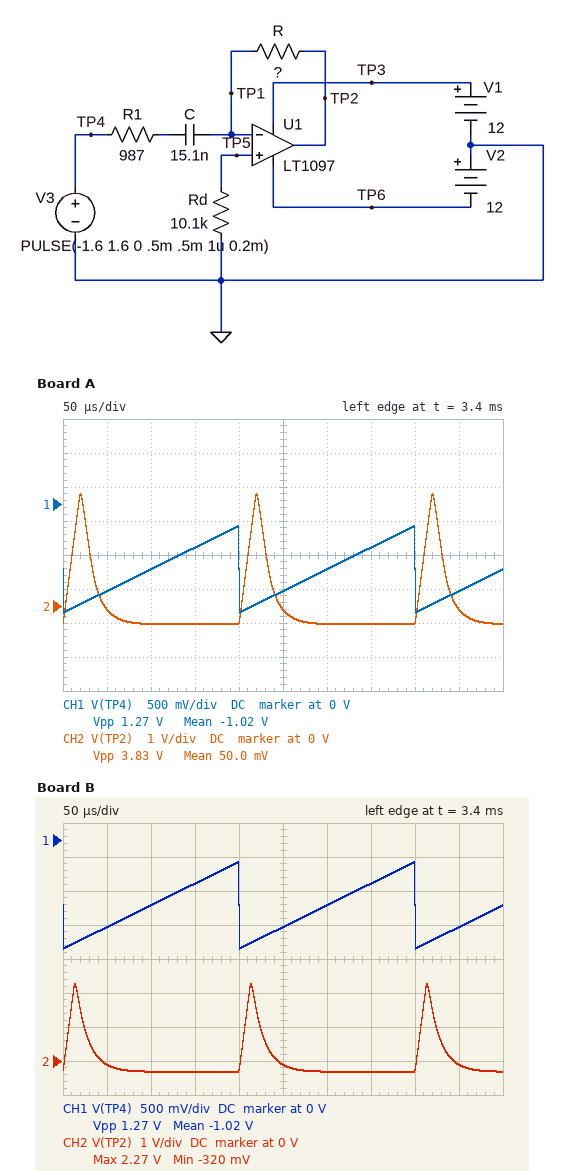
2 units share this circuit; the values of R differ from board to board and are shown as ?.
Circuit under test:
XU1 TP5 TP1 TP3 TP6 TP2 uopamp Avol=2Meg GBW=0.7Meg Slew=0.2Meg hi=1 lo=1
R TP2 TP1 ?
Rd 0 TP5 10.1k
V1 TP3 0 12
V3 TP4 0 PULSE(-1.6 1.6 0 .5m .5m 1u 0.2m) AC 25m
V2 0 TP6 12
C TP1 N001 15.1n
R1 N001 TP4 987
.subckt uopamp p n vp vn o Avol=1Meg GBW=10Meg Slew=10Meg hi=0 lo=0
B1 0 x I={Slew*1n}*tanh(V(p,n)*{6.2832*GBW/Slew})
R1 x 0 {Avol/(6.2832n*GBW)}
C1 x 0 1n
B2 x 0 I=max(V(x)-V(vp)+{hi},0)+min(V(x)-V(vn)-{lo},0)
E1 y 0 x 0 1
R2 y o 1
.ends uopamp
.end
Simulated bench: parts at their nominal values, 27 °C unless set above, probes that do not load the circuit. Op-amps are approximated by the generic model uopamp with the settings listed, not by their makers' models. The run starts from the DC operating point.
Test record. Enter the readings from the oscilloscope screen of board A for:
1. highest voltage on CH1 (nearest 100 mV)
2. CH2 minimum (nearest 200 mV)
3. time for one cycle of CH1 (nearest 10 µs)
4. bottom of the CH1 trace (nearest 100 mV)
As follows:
-300 mV
-600 mV
200 µs
-1.6 V
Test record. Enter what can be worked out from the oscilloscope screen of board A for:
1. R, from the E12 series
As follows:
5.6 kΩ
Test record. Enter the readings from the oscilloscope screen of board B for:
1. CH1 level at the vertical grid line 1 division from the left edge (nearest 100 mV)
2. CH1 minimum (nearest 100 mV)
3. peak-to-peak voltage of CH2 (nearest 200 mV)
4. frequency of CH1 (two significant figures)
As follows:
-1.3 V
-1.6 V
2.6 V
5.0 kHz
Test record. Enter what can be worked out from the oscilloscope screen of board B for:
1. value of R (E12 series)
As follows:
3.3 kΩ
